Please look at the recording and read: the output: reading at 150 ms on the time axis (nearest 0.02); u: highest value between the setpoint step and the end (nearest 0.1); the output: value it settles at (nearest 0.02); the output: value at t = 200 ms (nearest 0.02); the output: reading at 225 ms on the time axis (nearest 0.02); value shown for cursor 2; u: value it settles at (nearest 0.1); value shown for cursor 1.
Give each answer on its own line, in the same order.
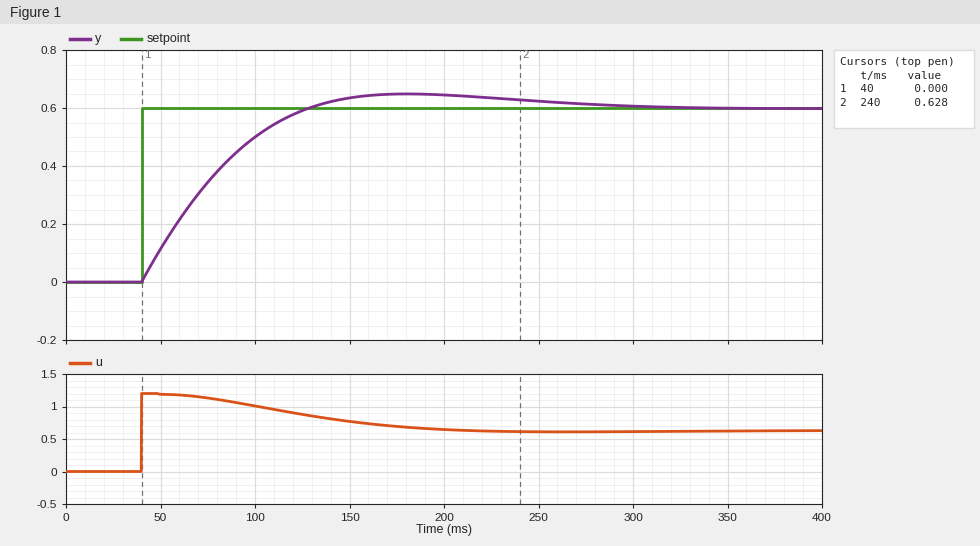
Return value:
0.64
1.2
0.60
0.64
0.64
0.628
0.6
0.000
